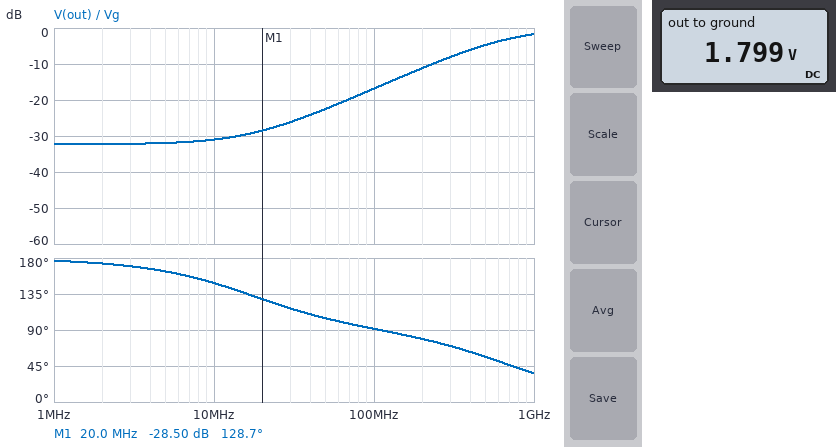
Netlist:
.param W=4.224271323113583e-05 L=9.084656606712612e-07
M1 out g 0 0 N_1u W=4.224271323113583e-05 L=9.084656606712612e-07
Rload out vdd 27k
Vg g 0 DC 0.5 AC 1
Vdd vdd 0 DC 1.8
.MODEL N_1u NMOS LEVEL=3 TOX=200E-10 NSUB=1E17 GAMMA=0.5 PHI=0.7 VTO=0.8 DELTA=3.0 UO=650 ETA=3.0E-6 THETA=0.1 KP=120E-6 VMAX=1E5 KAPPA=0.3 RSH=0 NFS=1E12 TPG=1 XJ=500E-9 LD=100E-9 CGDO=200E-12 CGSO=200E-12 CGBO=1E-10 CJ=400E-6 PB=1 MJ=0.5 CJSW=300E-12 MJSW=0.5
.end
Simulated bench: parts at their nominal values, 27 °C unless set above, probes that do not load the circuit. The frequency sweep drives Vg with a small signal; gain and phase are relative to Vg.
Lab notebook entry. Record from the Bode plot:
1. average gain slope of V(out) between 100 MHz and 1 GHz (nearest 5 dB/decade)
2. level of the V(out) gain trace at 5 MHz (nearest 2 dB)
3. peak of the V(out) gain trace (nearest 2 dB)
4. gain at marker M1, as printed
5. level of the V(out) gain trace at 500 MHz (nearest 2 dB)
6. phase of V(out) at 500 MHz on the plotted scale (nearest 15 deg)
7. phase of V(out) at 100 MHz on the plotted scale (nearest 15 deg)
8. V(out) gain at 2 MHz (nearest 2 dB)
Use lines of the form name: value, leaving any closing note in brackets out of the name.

average gain slope of V(out) between 100 MHz and 1 GHz: 15 dB/decade
level of the V(out) gain trace at 5 MHz: -32 dB
peak of the V(out) gain trace: -2 dB
gain at marker M1, as printed: -28.50 dB
level of the V(out) gain trace at 500 MHz: -4 dB
phase of V(out) at 500 MHz on the plotted scale: 60 deg
phase of V(out) at 100 MHz on the plotted scale: 90 deg
V(out) gain at 2 MHz: -32 dB
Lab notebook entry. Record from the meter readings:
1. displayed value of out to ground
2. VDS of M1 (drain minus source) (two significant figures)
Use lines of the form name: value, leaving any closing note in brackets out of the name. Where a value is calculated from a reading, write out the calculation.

displayed value of out to ground: 1.799 V
VDS of M1 (drain minus source): 1.799 V = 1.8 V
